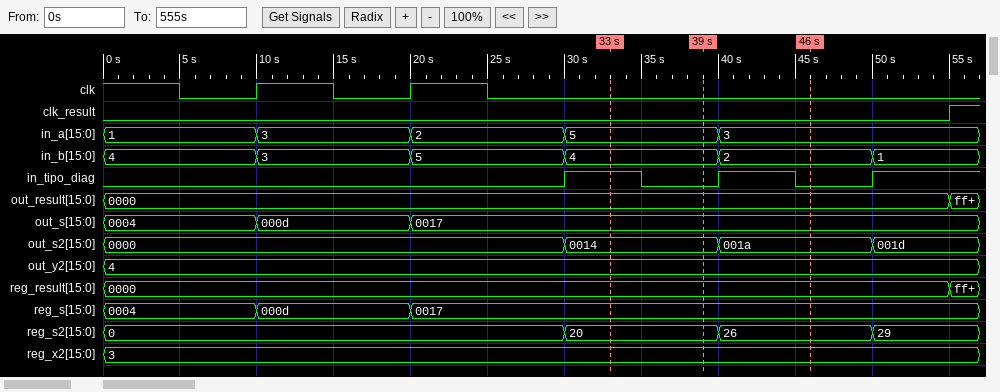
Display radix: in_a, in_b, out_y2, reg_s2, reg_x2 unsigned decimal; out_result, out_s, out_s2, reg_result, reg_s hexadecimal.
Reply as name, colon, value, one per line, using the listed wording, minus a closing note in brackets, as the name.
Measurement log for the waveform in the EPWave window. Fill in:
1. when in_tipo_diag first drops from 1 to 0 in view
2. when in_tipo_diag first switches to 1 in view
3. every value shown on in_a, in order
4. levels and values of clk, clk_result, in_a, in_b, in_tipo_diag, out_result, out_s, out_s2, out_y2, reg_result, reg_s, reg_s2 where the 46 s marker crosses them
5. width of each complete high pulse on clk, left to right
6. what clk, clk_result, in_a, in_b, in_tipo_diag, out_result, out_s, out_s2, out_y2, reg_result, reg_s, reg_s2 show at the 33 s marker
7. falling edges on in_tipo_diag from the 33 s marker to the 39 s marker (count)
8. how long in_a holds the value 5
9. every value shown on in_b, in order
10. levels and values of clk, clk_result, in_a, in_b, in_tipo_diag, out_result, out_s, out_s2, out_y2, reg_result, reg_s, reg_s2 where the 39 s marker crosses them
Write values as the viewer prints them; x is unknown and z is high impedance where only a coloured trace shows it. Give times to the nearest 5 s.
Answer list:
when in_tipo_diag first drops from 1 to 0 in view: 35 s
when in_tipo_diag first switches to 1 in view: 30 s
every value shown on in_a, in order: 1, 3, 2, 5, 3
levels and values of clk, clk_result, in_a, in_b, in_tipo_diag, out_result, out_s, out_s2, out_y2, reg_result, reg_s, reg_s2 where the 46 s marker crosses them: clk=0, clk_result=0, in_a=3, in_b=2, in_tipo_diag=0, out_result=0000, out_s=0017, out_s2=001a, out_y2=4, reg_result=0000, reg_s=0017, reg_s2=26
width of each complete high pulse on clk, left to right: 5 s, 5 s
what clk, clk_result, in_a, in_b, in_tipo_diag, out_result, out_s, out_s2, out_y2, reg_result, reg_s, reg_s2 show at the 33 s marker: clk=0, clk_result=0, in_a=5, in_b=4, in_tipo_diag=1, out_result=0000, out_s=0017, out_s2=0014, out_y2=4, reg_result=0000, reg_s=0017, reg_s2=20
falling edges on in_tipo_diag from the 33 s marker to the 39 s marker: 1
how long in_a holds the value 5: 10 s
every value shown on in_b, in order: 4, 3, 5, 4, 2, 1
levels and values of clk, clk_result, in_a, in_b, in_tipo_diag, out_result, out_s, out_s2, out_y2, reg_result, reg_s, reg_s2 where the 39 s marker crosses them: clk=0, clk_result=0, in_a=5, in_b=4, in_tipo_diag=0, out_result=0000, out_s=0017, out_s2=0014, out_y2=4, reg_result=0000, reg_s=0017, reg_s2=20
